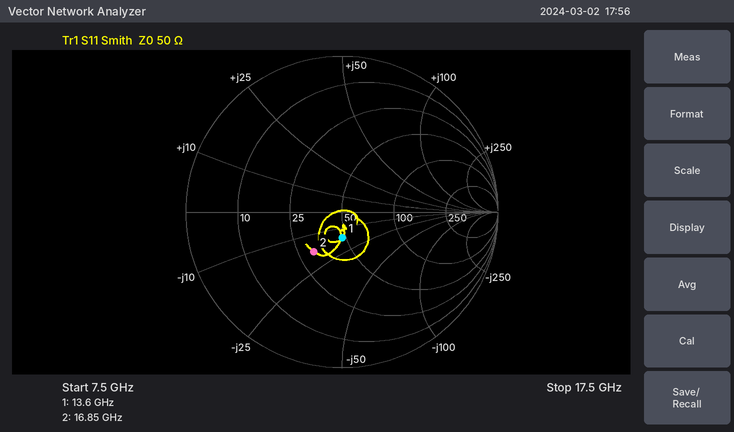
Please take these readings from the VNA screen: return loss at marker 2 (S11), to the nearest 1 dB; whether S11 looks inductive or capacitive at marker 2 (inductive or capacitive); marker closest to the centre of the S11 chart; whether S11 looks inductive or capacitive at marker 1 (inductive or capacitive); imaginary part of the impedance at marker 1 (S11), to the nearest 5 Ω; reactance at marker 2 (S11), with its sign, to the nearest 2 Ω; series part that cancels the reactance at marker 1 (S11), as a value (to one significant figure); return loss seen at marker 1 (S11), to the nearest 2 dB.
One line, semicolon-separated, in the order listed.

10 dB; capacitive; marker 1; capacitive; -15 Ω; -18 Ω; 200 pH; 16 dB
